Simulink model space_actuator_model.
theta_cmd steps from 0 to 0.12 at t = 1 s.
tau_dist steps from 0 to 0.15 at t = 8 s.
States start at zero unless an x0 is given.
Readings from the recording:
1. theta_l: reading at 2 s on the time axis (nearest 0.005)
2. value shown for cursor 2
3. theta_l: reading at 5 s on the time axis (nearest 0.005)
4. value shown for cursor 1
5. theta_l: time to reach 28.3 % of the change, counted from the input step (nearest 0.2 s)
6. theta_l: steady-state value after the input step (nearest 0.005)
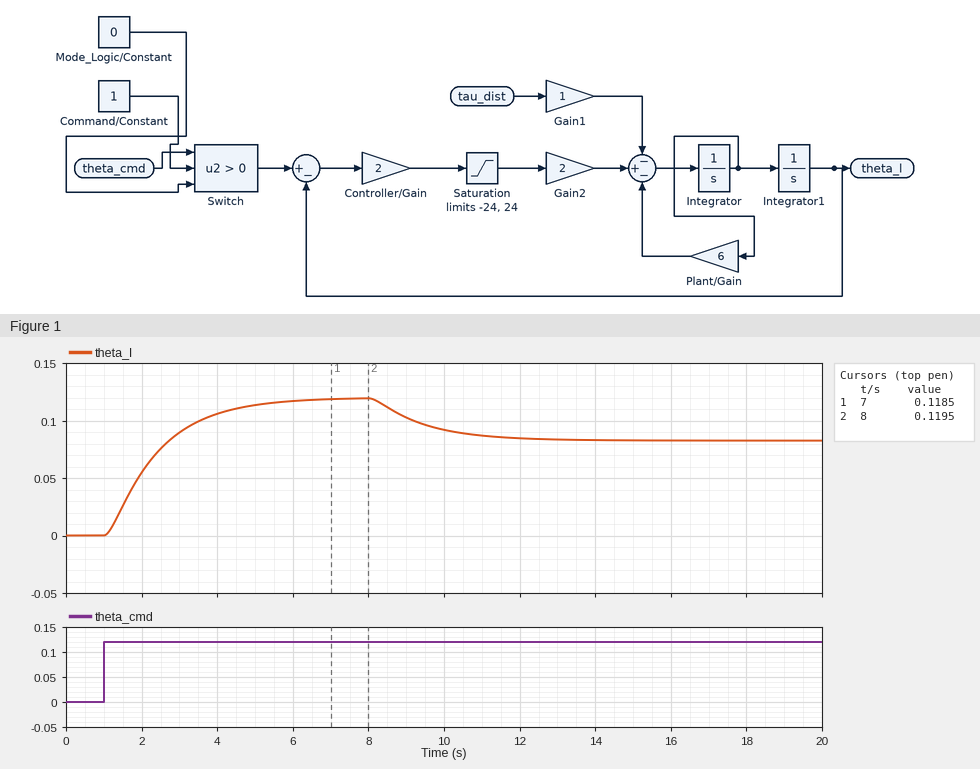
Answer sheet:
0.055
0.1195
0.115
0.1185
0.6 s
0.120
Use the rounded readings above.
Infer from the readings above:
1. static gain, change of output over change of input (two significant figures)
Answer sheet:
1.0
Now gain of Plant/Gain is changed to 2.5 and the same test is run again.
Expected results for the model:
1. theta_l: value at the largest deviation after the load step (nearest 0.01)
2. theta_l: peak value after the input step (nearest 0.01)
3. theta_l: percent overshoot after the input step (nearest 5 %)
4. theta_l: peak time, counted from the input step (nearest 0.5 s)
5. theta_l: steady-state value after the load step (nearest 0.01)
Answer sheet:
0.08
0.13
10 %
2.0 s
0.08
